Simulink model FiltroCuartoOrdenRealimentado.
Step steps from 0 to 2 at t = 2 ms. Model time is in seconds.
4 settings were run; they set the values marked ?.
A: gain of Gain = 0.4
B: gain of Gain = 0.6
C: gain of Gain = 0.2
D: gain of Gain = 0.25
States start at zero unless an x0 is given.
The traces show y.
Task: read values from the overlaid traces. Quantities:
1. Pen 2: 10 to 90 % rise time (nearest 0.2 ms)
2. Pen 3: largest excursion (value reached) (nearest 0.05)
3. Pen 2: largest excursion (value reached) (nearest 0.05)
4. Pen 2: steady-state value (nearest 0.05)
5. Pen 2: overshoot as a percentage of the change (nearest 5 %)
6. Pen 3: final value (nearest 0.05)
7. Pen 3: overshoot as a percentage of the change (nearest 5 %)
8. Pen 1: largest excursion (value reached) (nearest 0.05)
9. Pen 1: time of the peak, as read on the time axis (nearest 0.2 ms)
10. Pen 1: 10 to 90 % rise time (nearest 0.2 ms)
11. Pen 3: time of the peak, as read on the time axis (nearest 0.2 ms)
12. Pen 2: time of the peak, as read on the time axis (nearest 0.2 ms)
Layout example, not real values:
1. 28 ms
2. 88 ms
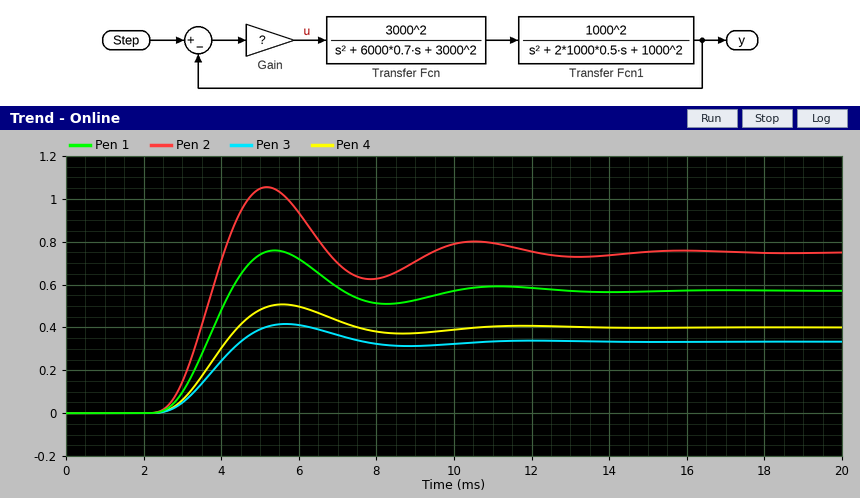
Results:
1. 1.2 ms
2. 0.40
3. 1.05
4. 0.75
5. 40 %
6. 0.35
7. 25 %
8. 0.75
9. 5.4 ms
10. 1.2 ms
11. 5.6 ms
12. 5.2 ms
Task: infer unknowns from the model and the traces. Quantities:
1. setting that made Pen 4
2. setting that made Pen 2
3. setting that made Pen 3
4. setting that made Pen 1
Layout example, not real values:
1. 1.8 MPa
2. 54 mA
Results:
1. D
2. B
3. C
4. A
